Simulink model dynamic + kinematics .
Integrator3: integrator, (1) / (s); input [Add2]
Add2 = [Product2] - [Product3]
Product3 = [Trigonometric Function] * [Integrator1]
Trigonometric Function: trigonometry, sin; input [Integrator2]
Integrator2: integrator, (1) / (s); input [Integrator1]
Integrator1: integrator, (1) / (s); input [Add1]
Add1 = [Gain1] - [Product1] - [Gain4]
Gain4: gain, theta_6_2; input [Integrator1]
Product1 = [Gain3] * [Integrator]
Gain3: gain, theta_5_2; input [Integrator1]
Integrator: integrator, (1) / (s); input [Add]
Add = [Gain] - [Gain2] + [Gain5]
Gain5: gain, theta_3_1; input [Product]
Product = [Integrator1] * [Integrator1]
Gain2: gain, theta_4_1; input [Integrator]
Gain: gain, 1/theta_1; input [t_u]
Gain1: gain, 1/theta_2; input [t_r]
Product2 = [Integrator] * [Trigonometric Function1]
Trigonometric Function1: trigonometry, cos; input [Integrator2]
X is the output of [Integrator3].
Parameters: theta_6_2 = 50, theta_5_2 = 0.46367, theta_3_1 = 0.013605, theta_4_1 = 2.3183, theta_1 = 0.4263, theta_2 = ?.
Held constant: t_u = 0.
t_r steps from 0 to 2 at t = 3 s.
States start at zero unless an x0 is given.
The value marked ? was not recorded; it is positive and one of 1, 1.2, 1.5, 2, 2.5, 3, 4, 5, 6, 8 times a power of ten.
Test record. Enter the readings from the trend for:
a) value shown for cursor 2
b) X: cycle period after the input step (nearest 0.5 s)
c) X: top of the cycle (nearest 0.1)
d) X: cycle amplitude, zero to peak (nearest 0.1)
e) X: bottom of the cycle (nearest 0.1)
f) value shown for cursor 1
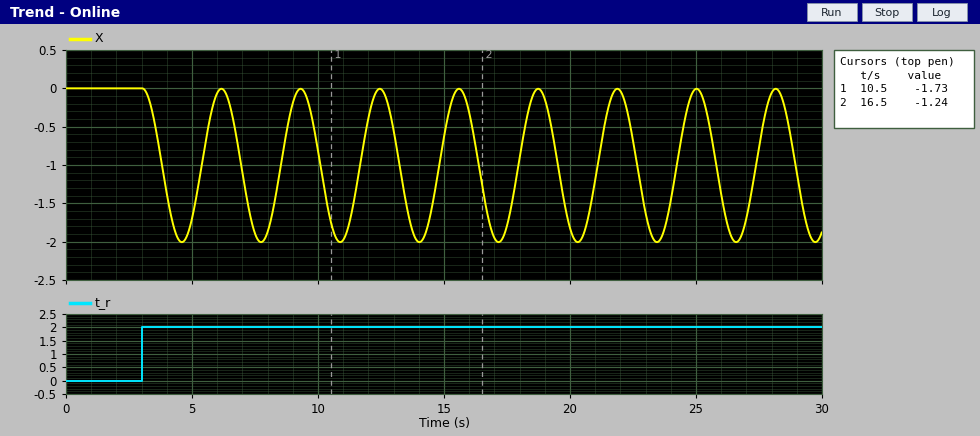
-1.24
3.0 s
0.0
1.0
-2.0
-1.73
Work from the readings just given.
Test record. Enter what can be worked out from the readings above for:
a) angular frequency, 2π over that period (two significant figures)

2.1 rad/s
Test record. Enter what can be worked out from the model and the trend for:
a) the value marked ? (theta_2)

0.02
